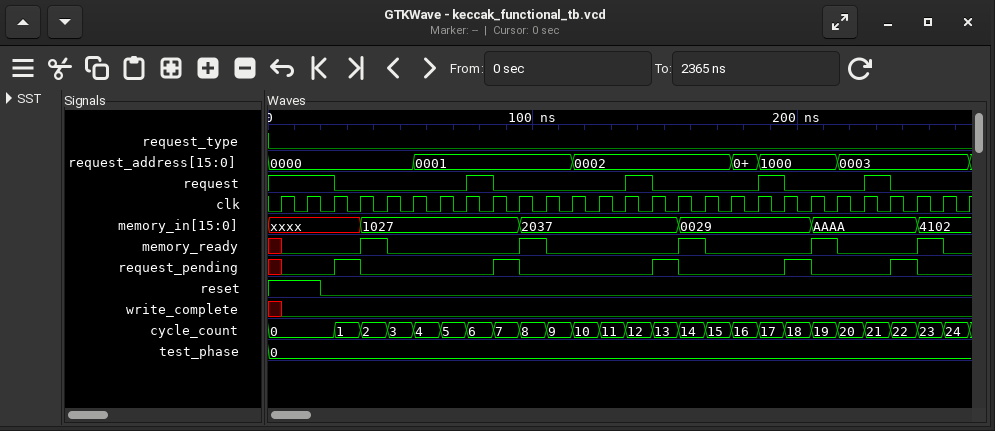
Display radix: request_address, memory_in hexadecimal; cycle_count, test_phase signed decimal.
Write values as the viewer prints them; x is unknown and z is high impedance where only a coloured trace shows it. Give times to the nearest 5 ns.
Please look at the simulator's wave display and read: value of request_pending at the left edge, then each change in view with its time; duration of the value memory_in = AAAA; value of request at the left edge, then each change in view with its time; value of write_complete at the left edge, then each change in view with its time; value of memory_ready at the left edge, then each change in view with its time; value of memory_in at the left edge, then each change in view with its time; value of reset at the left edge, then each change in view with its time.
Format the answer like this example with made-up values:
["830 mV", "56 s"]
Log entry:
["x, 0 at 5 ns, 1 at 25 ns, 0 at 35 ns, 1 at 85 ns, 0 at 95 ns, 1 at 145 ns, 0 at 155 ns, 1 at 195 ns, 0 at 205 ns, 1 at 235 ns, 0 at 245 ns", "40 ns", "1, 0 at 25 ns, 1 at 75 ns, 0 at 85 ns, 1 at 135 ns, 0 at 145 ns, 1 at 185 ns, 0 at 195 ns, 1 at 225 ns, 0 at 235 ns", "x, 0 at 5 ns", "x, 0 at 5 ns, 1 at 35 ns, 0 at 45 ns, 1 at 95 ns, 0 at 105 ns, 1 at 155 ns, 0 at 165 ns, 1 at 205 ns, 0 at 215 ns, 1 at 245 ns, 0 at 255 ns", "xxxx, 1027 at 35 ns, 2037 at 95 ns, 0029 at 155 ns, AAAA at 205 ns, 4102 at 245 ns", "1, 0 at 20 ns"]
